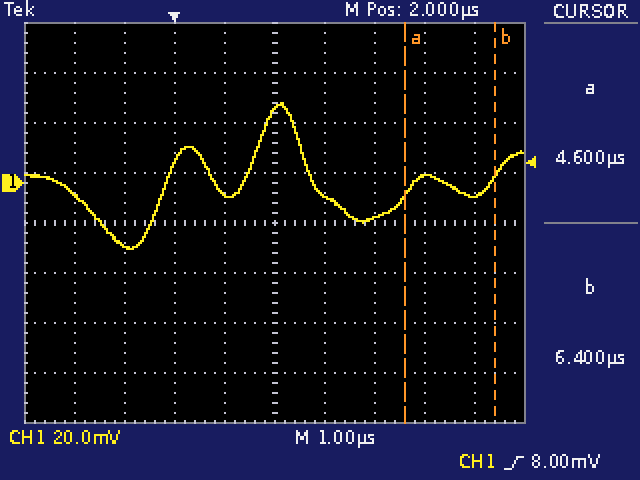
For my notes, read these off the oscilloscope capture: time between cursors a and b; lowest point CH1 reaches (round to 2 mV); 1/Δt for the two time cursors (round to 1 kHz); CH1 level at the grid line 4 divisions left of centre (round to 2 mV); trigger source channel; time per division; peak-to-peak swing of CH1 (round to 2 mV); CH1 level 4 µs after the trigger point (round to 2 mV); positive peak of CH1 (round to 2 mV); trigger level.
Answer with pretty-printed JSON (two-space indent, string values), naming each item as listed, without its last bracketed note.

{
  "time between cursors a and b": "1.8 µs",
  "lowest point CH1 reaches": "-26 mV",
  "1/Δt for the two time cursors": "556 kHz",
  "CH1 level at the grid line 4 divisions left of centre": "-4 mV",
  "trigger source channel": "CH1",
  "time per division": "1 µs",
  "peak-to-peak swing of CH1": "58 mV",
  "CH1 level 4 µs after the trigger point": "-14 mV",
  "positive peak of CH1": "32 mV",
  "trigger level": "8.00 mV"
}
